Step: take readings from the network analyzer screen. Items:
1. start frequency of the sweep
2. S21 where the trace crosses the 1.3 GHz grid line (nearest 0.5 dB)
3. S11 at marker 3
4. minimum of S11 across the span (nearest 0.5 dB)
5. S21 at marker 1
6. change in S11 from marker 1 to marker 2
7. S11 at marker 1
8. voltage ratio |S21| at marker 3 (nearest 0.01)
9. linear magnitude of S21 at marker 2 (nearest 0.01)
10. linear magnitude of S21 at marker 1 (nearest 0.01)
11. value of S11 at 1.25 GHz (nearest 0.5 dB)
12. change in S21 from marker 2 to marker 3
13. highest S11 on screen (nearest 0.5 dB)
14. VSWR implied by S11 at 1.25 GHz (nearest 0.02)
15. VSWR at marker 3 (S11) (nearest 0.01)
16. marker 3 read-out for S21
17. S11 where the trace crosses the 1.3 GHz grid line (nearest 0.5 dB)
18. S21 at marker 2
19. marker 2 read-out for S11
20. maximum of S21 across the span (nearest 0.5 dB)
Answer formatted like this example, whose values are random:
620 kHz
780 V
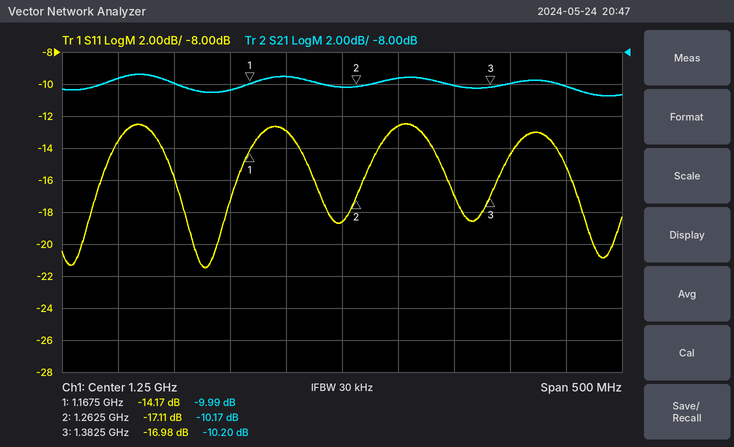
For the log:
1 GHz
-9.5 dB
-16.98 dB
-21.5 dB
-9.99 dB
-2.94 dB
-14.17 dB
0.31
0.31
0.32
-18.5 dB
-0.03 dB
-12.5 dB
1.26
1.33
-10.20 dB
-12.5 dB
-10.17 dB
-17.11 dB
-9.5 dB
